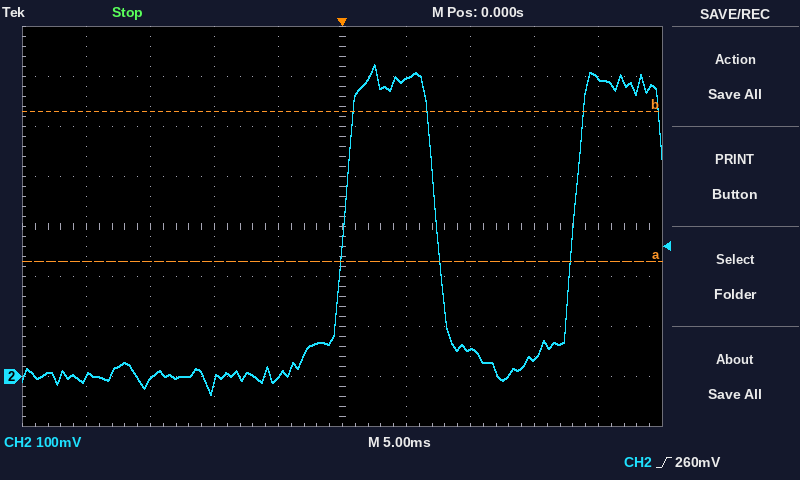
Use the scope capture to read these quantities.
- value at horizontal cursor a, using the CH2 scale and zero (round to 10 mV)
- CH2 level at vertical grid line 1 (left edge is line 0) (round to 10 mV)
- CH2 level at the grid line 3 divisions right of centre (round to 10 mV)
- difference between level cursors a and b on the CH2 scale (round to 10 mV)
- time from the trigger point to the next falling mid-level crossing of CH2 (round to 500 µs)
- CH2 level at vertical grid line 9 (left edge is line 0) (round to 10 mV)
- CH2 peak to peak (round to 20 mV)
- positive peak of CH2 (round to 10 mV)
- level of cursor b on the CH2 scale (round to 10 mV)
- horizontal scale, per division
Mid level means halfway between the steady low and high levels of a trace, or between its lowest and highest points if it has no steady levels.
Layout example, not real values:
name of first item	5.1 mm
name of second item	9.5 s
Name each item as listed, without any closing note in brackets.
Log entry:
value at horizontal cursor a, using the CH2 scale and zero	230 mV
CH2 level at vertical grid line 1 (left edge is line 0)	0 mV
CH2 level at the grid line 3 divisions right of centre	40 mV
difference between level cursors a and b on the CH2 scale	300 mV
time from the trigger point to the next falling mid-level crossing of CH2	7.5 ms
CH2 level at vertical grid line 9 (left edge is line 0)	600 mV
CH2 peak to peak	660 mV
positive peak of CH2	620 mV
level of cursor b on the CH2 scale	530 mV
horizontal scale, per division	5 ms
